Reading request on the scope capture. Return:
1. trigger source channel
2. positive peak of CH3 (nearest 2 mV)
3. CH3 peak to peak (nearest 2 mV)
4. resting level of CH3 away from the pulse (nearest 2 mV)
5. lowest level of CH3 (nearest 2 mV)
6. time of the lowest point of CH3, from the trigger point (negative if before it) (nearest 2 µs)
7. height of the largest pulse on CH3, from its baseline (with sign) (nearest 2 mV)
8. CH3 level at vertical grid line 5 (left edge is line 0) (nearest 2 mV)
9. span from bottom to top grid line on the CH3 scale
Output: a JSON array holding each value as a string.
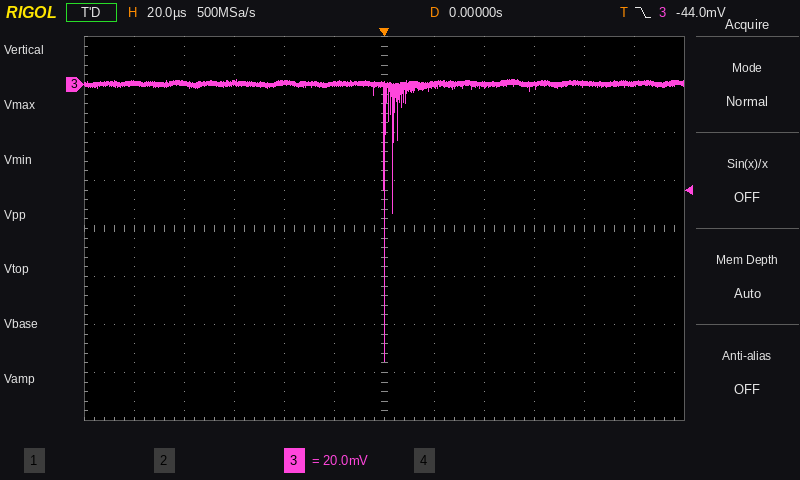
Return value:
["CH3", "2 mV", "118 mV", "0 mV", "-116 mV", "0 µs", "-116 mV", "0 mV", "160 mV"]
